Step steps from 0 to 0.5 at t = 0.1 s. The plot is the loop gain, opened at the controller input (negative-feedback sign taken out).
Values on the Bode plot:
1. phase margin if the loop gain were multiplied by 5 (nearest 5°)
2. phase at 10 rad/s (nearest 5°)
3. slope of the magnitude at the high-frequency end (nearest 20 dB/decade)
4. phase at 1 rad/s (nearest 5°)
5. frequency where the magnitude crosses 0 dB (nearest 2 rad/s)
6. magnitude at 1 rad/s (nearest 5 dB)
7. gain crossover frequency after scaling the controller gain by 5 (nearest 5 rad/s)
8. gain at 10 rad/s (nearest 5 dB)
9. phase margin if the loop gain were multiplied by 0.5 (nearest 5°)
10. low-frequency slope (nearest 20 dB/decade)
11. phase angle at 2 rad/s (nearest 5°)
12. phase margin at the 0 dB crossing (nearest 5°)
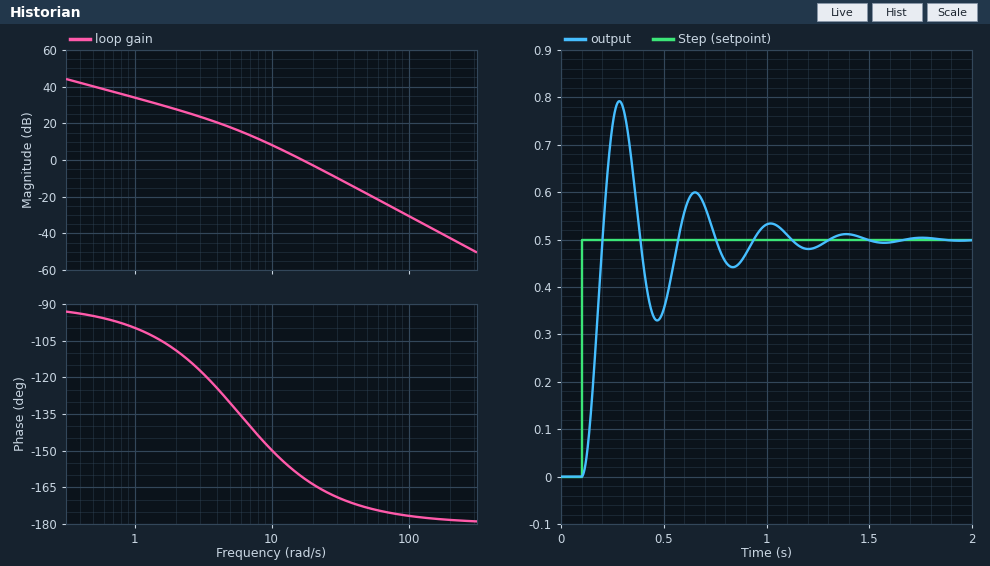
10°
-150°
-40 dB/decade
-100°
16 rad/s
35 dB
40 rad/s
10 dB
25°
-20 dB/decade
-110°
20°
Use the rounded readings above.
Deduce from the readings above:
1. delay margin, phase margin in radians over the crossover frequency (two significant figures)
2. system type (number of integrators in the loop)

0.022 s
1
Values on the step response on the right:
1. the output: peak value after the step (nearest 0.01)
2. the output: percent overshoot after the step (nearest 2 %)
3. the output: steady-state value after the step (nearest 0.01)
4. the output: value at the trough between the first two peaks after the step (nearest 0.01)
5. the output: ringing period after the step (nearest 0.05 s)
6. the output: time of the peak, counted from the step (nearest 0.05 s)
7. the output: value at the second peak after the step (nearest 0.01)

0.79
58 %
0.50
0.33
0.35 s
0.20 s
0.60
